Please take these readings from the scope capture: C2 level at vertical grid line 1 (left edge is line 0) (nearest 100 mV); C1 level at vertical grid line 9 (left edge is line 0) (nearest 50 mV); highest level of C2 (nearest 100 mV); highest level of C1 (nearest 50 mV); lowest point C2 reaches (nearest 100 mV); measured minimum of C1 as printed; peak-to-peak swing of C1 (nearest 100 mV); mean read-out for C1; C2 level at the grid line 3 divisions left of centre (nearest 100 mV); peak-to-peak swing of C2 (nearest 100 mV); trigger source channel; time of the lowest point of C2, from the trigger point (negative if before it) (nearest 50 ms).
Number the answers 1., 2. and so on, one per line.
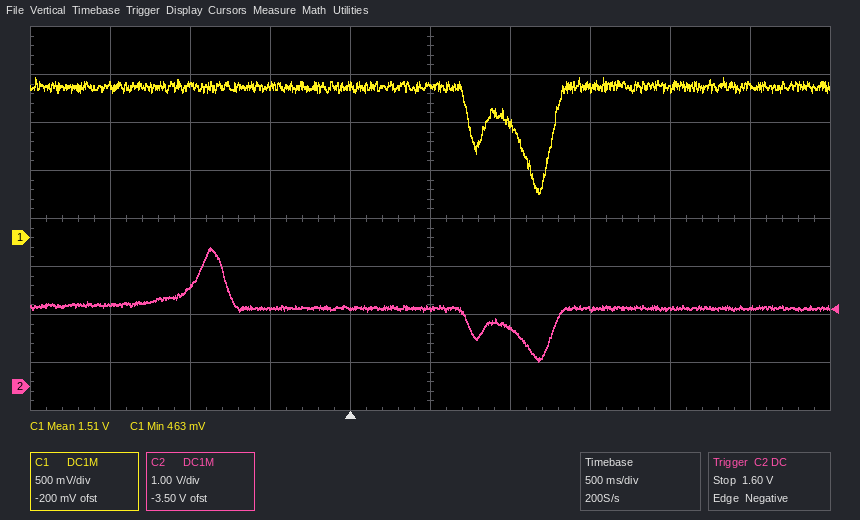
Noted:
1. 1.7 V
2. 1.60 V
3. 2.9 V
4. 1.65 V
5. 500 mV
6. 463 mV
7. 1.20 V
8. 1.51 V
9. 2.1 V
10. 2.4 V
11. C2
12. +1.20 s
